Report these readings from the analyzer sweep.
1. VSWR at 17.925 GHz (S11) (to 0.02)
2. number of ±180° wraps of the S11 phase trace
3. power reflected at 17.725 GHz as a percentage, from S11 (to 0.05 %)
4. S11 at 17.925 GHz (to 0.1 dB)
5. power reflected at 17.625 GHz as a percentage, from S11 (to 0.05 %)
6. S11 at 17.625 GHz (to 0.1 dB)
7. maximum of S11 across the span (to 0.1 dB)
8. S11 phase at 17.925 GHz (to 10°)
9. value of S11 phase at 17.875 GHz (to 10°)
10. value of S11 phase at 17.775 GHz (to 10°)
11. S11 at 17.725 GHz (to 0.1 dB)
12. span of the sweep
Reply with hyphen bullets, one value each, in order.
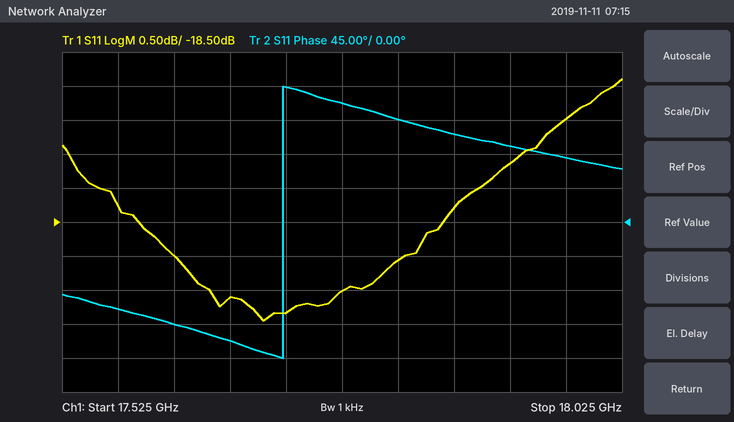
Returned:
- 1.30
- 1
- 1.05 %
- -17.6 dB
- 1.25 %
- -19.0 dB
- -16.4 dB
- 100°
- 120°
- 160°
- -19.8 dB
- 500 MHz
